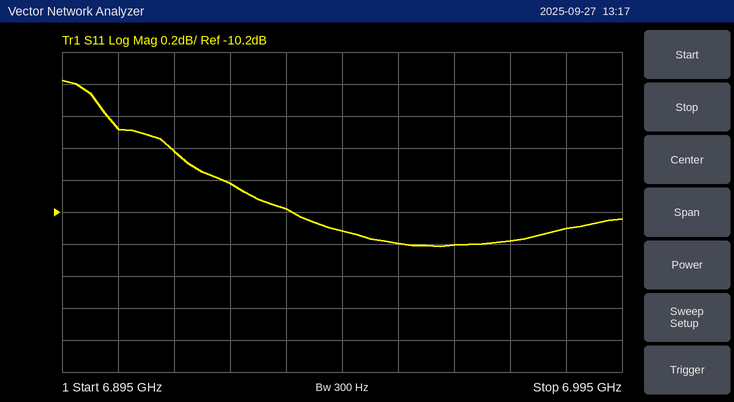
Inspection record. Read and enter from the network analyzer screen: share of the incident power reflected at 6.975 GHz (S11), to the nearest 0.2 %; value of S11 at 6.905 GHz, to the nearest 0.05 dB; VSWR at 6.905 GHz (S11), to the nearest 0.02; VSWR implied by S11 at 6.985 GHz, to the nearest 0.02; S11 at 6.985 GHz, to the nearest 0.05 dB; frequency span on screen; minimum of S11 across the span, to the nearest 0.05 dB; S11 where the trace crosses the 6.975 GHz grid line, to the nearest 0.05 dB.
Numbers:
9.2 %
-9.70 dB
1.98
1.88
-10.30 dB
100 MHz
-10.40 dB
-10.40 dB
